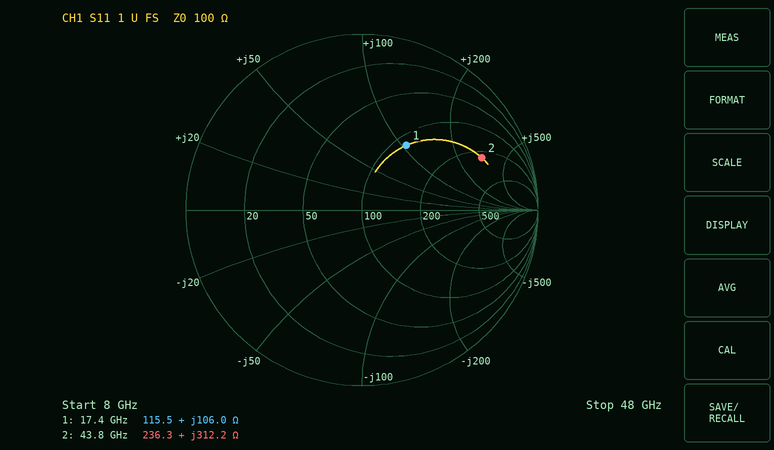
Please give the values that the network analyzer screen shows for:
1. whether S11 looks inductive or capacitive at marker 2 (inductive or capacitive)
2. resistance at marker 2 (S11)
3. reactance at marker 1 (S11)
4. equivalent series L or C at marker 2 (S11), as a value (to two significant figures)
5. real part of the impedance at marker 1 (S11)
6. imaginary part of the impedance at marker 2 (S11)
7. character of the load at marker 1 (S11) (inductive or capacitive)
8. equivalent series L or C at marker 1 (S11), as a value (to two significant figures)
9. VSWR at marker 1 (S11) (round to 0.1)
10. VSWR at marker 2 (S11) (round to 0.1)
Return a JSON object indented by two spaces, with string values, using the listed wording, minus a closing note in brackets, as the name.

{
  "whether S11 looks inductive or capacitive at marker 2": "inductive",
  "resistance at marker 2": "236.3 Ω",
  "reactance at marker 1": "+106.0 Ω",
  "equivalent series L or C at marker 2 (S11), as a value": "1.1 nH",
  "real part of the impedance at marker 1": "115.5 Ω",
  "imaginary part of the impedance at marker 2": "+312.2 Ω",
  "character of the load at marker 1 (S11)": "inductive",
  "equivalent series L or C at marker 1 (S11), as a value": "970 pH",
  "VSWR at marker 1 (S11)": "2.6",
  "VSWR at marker 2 (S11)": "6.8"
}
